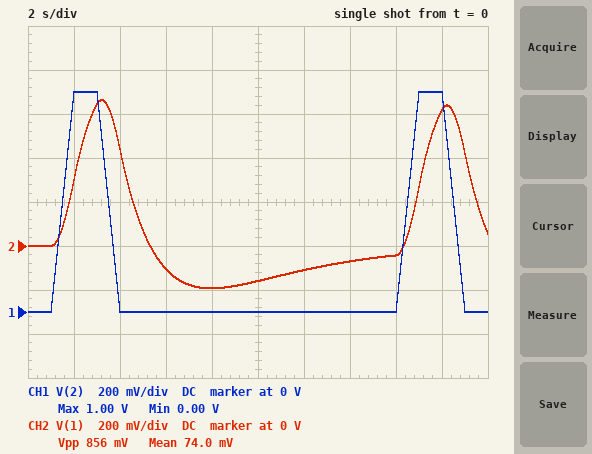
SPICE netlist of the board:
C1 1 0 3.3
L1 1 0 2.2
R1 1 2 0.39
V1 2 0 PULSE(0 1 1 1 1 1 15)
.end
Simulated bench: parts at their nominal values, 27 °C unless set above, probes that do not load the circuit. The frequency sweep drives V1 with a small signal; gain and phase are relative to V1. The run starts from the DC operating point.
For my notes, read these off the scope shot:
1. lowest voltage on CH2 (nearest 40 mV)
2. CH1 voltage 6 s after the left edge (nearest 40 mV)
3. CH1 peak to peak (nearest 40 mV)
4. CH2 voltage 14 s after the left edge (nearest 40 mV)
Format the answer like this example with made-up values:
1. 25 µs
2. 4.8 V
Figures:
1. -200 mV
2. 0 V
3. 1.00 V
4. -80 mV
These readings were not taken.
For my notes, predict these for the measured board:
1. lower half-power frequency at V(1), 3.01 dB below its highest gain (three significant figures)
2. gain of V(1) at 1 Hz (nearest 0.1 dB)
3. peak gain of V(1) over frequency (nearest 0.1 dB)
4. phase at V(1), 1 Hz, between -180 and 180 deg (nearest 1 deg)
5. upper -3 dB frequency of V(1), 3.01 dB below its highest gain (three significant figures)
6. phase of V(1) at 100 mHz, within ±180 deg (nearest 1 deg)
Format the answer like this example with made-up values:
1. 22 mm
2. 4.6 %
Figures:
1. 23.7 mHz
2. -18.2 dB
3. 0 dB
4. -83 deg
5. 147 mHz
6. -28 deg
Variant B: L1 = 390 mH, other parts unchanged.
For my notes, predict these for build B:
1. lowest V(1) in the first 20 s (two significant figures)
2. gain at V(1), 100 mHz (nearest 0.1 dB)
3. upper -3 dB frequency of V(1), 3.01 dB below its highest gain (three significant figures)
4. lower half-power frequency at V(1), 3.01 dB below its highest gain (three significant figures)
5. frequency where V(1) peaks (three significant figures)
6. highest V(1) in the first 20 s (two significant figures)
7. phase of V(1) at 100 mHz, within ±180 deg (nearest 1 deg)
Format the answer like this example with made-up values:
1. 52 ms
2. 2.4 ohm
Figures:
1. -440 mV
2. -2.1 dB
3. 215 mHz
4. 91.5 mHz
5. 140 mHz
6. 500 mV
7. 38 deg
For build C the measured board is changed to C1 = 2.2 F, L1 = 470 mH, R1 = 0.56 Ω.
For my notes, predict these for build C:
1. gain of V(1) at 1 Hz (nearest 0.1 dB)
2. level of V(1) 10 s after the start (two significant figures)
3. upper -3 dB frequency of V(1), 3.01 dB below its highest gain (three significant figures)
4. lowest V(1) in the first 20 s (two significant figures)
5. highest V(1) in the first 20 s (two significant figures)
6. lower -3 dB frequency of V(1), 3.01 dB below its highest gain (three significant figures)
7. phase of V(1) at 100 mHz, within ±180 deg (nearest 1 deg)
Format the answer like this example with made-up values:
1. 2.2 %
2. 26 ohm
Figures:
1. -17.6 dB
2. 57 mV
3. 234 mHz
4. -470 mV
5. 470 mV
6. 105 mHz
7. 48 deg
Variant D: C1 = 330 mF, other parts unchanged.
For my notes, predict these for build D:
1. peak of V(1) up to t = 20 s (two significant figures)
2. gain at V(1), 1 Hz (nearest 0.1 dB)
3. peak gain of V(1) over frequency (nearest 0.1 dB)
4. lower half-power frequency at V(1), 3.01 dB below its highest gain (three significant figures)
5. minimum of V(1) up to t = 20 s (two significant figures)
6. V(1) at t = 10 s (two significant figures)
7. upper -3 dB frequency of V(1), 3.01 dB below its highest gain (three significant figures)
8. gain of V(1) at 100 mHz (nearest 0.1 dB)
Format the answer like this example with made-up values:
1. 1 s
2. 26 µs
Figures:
1. 900 mV
2. -2.1 dB
3. 0 dB
4. 27.6 mHz
5. -280 mV
6. -98 mV
7. 1.26 Hz
8. -0.2 dB
